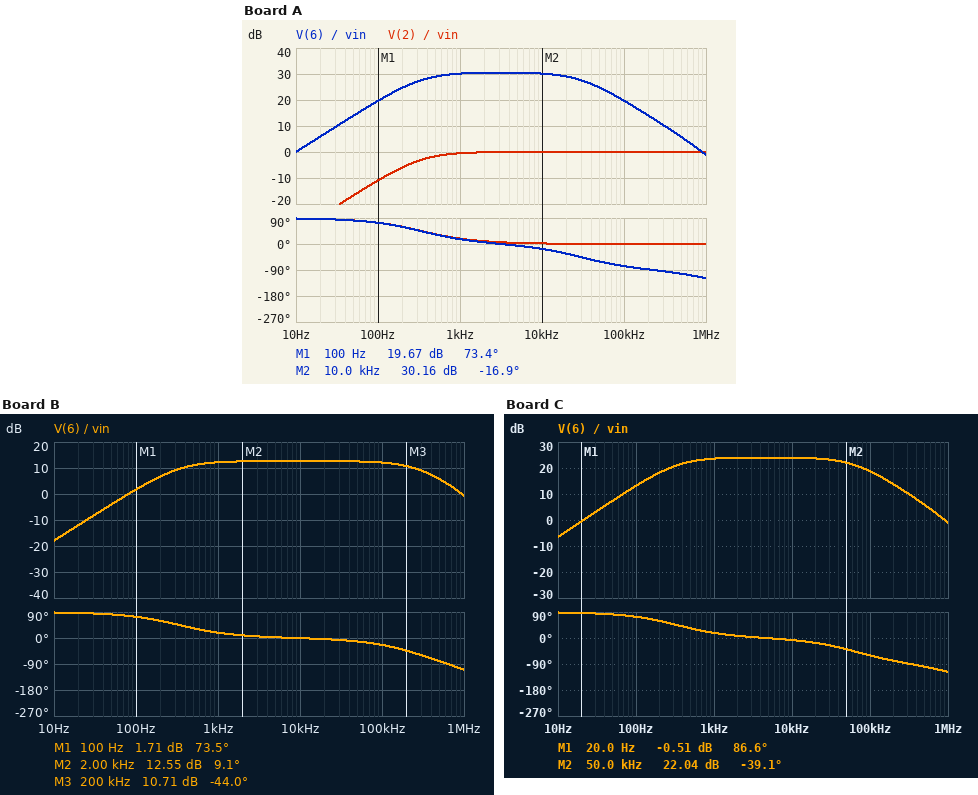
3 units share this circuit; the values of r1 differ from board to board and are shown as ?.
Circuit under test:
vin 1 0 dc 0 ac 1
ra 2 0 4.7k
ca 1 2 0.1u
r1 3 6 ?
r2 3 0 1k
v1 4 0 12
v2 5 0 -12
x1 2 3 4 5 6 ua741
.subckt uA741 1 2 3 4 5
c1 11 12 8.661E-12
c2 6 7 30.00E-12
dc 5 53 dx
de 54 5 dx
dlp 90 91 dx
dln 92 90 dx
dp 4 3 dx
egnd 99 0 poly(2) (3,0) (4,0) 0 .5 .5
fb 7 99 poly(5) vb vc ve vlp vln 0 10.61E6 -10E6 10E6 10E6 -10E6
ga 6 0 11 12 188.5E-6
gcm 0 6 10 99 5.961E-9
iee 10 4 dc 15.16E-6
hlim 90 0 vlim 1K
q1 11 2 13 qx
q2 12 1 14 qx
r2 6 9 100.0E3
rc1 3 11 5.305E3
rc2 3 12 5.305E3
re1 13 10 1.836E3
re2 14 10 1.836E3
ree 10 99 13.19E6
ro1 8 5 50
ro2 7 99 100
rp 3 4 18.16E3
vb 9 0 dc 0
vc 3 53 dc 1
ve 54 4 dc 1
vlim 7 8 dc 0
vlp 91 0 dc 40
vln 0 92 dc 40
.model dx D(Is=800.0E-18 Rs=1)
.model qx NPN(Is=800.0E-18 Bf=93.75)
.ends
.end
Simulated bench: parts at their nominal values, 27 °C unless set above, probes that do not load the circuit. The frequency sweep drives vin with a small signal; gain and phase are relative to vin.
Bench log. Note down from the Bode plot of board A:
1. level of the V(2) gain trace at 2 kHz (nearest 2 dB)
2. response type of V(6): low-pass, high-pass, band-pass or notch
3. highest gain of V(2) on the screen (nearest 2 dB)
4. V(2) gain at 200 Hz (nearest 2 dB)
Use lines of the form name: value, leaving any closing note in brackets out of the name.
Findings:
level of the V(2) gain trace at 2 kHz: 0 dB
response type of V(6): low-pass, high-pass, band-pass or notch: band-pass
highest gain of V(2) on the screen: 0 dB
V(2) gain at 200 Hz: -6 dB
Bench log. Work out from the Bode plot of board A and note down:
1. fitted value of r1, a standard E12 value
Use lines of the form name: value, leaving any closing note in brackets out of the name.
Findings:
fitted value of r1, a standard E12 value: 33 kΩ
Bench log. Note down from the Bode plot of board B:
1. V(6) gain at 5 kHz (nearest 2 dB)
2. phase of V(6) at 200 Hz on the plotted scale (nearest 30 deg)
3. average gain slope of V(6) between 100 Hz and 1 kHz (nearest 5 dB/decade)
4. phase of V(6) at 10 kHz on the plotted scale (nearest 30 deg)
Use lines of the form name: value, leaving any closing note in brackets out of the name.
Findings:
V(6) gain at 5 kHz: 12 dB
phase of V(6) at 200 Hz on the plotted scale: 60 deg
average gain slope of V(6) between 100 Hz and 1 kHz: 10 dB/decade
phase of V(6) at 10 kHz on the plotted scale: 0 deg
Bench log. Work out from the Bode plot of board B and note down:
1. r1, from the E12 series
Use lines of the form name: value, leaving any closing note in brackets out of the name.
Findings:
r1, from the E12 series: 3.3 kΩ
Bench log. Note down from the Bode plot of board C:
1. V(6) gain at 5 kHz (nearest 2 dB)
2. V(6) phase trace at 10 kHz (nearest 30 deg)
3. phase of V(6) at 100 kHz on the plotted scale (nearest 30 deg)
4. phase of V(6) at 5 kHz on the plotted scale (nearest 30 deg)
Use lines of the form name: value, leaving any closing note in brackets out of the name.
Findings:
V(6) gain at 5 kHz: 24 dB
V(6) phase trace at 10 kHz: 0 deg
phase of V(6) at 100 kHz on the plotted scale: -60 deg
phase of V(6) at 5 kHz on the plotted scale: 0 deg
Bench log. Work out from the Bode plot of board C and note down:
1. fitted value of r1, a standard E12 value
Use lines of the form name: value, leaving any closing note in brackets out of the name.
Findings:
fitted value of r1, a standard E12 value: 15 kΩ
